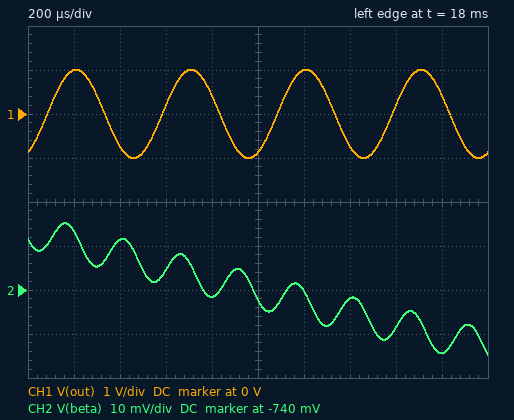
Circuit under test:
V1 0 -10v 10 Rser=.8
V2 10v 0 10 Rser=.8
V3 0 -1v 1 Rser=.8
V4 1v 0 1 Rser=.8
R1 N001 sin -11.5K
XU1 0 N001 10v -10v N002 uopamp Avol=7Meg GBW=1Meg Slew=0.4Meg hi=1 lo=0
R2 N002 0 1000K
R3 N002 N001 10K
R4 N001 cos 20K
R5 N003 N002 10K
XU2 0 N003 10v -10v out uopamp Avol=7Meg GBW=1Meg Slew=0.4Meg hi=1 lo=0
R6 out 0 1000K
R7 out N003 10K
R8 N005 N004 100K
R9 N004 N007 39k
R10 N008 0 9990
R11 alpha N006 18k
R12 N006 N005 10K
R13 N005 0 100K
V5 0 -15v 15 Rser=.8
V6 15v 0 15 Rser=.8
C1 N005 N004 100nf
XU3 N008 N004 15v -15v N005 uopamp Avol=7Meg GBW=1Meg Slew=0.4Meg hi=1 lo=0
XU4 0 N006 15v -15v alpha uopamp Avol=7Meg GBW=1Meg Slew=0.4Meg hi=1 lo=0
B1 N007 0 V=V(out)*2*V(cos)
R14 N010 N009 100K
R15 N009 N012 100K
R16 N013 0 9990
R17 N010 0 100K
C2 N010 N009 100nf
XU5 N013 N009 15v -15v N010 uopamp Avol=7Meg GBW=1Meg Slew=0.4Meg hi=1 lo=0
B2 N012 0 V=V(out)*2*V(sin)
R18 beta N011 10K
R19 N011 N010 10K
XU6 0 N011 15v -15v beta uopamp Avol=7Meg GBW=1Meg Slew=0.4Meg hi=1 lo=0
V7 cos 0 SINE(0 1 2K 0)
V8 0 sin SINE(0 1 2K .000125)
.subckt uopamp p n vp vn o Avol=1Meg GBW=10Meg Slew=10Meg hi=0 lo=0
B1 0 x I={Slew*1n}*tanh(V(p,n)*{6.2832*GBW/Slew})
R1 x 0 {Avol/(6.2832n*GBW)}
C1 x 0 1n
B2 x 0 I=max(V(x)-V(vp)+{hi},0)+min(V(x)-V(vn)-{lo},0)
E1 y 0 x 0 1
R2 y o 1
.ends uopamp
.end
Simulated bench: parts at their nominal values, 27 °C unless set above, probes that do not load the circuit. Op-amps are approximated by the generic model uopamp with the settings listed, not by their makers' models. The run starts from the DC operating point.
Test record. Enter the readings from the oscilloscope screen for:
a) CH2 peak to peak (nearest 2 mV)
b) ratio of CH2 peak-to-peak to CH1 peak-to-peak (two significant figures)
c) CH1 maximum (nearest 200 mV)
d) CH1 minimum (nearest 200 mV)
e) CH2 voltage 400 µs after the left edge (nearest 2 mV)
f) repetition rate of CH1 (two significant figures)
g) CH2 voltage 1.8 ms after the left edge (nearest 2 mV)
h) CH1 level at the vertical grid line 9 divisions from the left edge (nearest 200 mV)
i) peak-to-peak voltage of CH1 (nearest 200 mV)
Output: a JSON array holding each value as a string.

["30 mV", "0.015", "1.0 V", "-1.0 V", "-728 mV", "2.0 kHz", "-754 mV", "400 mV", "2.0 V"]
